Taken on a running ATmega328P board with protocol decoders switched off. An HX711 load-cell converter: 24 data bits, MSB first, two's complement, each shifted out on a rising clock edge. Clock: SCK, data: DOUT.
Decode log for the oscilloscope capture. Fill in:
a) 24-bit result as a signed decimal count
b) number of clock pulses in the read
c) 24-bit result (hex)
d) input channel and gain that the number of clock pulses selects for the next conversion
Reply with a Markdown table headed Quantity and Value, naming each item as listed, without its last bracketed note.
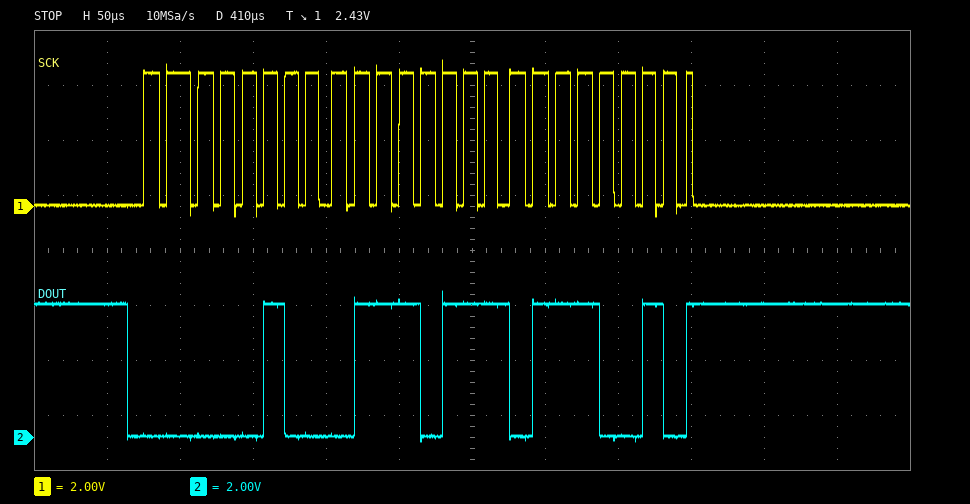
| Quantity | Value |
|---|---|
| 24-bit result as a signed decimal count | 292722 |
| number of clock pulses in the read | 25 |
| 24-bit result | 0x047772 |
| input channel and gain that the number of clock pulses selects for the next conversion | channel A, gain 128 |
